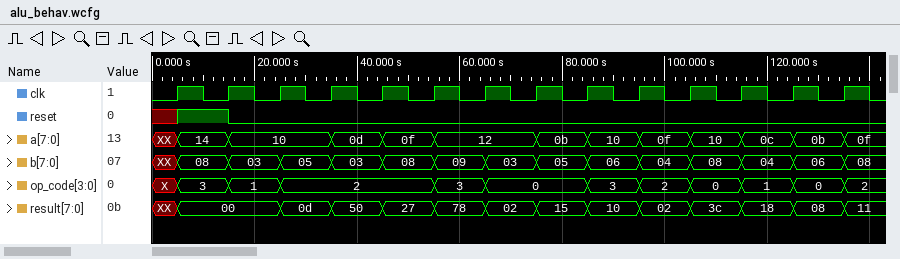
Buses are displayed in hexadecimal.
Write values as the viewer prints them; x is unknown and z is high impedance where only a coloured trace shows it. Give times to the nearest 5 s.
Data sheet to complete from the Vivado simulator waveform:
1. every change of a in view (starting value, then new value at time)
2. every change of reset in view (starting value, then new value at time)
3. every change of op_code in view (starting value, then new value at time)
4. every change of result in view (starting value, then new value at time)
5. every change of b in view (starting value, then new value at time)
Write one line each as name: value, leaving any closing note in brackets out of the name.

every change of a in view: XX, 14 at 5 s, 10 at 15 s, 0d at 35 s, 0f at 45 s, 12 at 55 s, 0b at 75 s, 10 at 85 s, 0f at 95 s, 10 at 105 s, 0c at 115 s, 0b at 125 s, 0f at 135 s
every change of reset in view: x, 1 at 5 s, 0 at 15 s
every change of op_code in view: X, 3 at 5 s, 1 at 15 s, 2 at 25 s, 3 at 55 s, 0 at 65 s, 3 at 85 s, 2 at 95 s, 0 at 105 s, 1 at 115 s, 0 at 125 s, 2 at 135 s
every change of result in view: XX, 00 at 5 s, 0d at 25 s, 50 at 35 s, 27 at 45 s, 78 at 55 s, 02 at 65 s, 15 at 75 s, 10 at 85 s, 02 at 95 s, 3c at 105 s, 18 at 115 s, 08 at 125 s, 11 at 135 s
every change of b in view: XX, 08 at 5 s, 03 at 15 s, 05 at 25 s, 03 at 35 s, 08 at 45 s, 09 at 55 s, 03 at 65 s, 05 at 75 s, 06 at 85 s, 04 at 95 s, 08 at 105 s, 04 at 115 s, 06 at 125 s, 08 at 135 s
